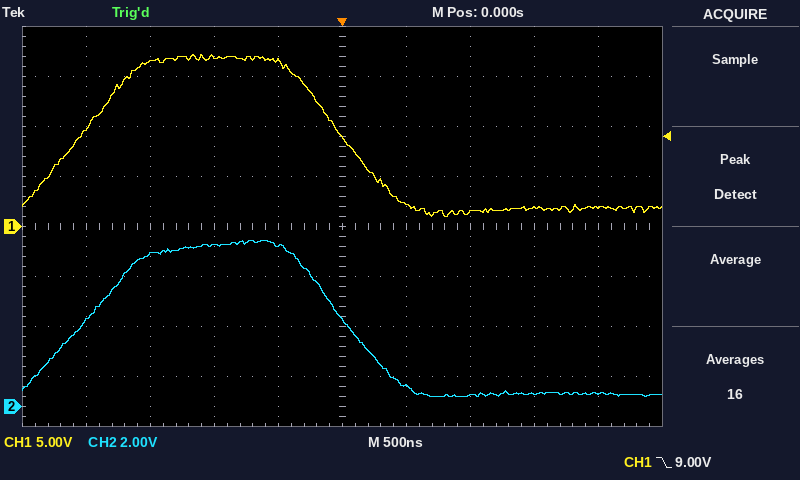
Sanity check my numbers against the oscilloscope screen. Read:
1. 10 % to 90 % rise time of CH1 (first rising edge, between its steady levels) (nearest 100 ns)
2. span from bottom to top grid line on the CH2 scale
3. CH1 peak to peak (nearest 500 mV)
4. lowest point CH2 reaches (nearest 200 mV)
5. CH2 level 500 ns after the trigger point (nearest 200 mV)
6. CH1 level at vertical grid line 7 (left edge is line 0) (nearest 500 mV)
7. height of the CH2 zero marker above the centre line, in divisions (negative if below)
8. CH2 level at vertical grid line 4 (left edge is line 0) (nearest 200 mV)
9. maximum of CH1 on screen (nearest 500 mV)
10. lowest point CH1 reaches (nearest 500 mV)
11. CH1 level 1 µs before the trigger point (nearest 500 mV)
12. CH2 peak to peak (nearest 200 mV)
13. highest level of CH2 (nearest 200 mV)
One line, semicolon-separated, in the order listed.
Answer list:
800 ns; 16 V; 16.0 V; 400 mV; 800 mV; 1.5 V; -3.6 div; 6.4 V; 17.0 V; 1.0 V; 17.0 V; 6.2 V; 6.6 V
